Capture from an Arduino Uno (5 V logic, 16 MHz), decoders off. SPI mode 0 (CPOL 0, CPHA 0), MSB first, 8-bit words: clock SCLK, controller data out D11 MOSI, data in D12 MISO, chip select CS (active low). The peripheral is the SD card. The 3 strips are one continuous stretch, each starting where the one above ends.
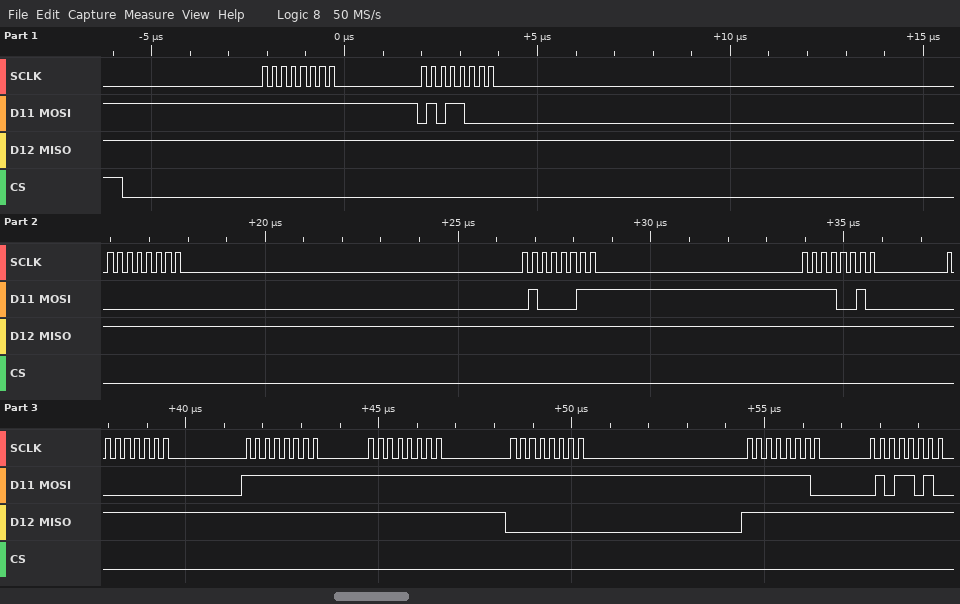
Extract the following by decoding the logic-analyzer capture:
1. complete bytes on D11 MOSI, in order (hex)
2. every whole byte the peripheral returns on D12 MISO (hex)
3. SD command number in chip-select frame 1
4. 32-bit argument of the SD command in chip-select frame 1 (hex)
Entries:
FF 58 00 43 F2 00 FF FF FF FE 5A
FF FF FF FF FF FF FF FF 00 FF FF
CMD24
0x0043F200
